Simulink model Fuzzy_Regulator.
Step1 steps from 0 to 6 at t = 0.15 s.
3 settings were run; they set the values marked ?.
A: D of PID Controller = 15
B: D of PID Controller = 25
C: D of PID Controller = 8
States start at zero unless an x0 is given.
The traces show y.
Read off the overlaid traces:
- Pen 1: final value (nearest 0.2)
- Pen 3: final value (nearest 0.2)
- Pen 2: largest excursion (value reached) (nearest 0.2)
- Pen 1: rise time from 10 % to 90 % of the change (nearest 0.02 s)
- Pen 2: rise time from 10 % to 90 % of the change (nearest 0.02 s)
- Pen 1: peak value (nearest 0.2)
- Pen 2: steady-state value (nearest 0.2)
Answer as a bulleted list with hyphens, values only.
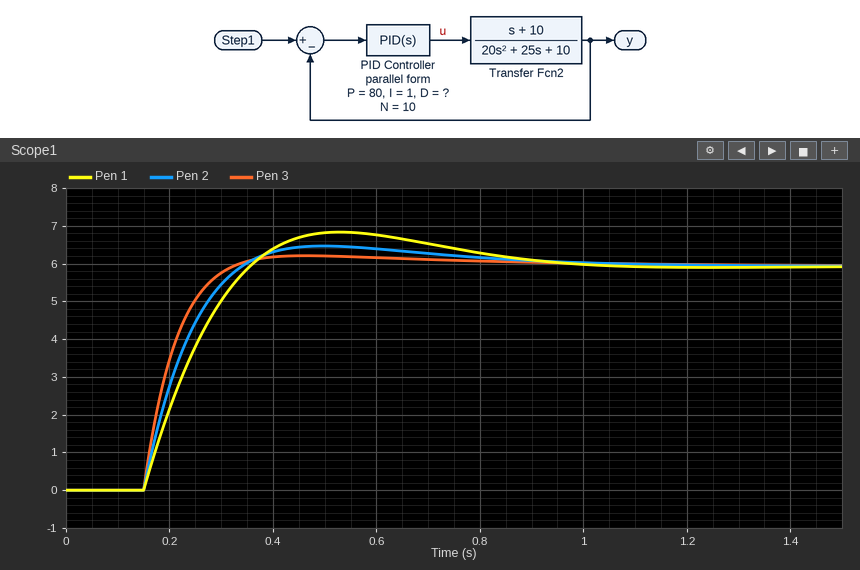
- 6.0
- 6.0
- 6.4
- 0.16 s
- 0.14 s
- 6.8
- 6.0
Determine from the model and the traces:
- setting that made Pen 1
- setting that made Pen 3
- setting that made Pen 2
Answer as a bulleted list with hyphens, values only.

- C
- B
- A
